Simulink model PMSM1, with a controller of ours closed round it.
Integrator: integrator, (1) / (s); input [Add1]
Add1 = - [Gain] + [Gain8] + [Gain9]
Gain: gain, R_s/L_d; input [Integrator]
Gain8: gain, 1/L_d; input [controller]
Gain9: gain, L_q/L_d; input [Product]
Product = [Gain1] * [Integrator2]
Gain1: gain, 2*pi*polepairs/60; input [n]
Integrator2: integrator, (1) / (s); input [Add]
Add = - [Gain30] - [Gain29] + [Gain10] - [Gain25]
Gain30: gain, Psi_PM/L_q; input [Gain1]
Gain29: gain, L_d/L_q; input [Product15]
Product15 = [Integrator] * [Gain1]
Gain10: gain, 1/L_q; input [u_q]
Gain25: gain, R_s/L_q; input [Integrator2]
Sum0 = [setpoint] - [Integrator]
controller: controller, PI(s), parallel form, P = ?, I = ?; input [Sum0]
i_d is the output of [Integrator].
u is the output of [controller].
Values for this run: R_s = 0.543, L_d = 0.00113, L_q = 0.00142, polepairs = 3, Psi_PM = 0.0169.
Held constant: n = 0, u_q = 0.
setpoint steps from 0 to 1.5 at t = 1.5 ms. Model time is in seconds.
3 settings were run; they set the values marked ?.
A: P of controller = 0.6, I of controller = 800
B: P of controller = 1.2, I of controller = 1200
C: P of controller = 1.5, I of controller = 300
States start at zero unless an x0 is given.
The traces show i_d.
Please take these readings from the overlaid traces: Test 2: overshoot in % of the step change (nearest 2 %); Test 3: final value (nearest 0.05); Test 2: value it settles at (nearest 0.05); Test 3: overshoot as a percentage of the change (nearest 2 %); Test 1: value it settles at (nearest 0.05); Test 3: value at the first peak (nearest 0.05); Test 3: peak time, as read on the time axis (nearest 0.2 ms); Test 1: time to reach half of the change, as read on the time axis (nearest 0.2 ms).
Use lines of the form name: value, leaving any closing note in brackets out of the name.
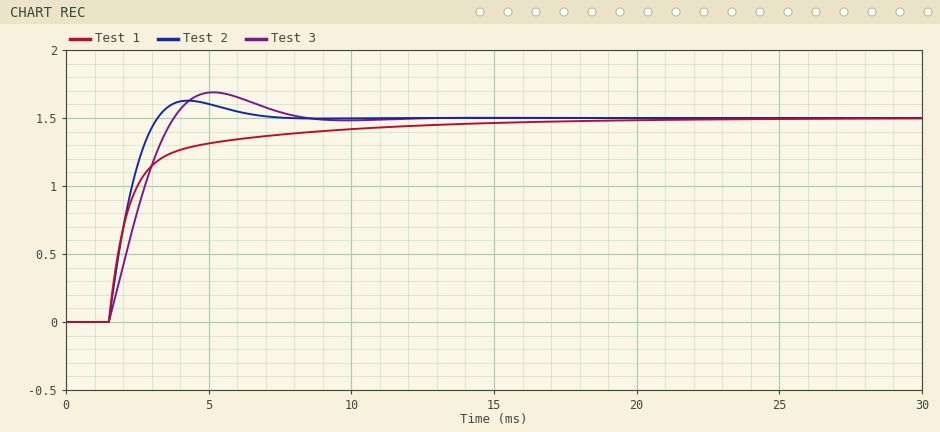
Test 2: overshoot in % of the step change: 8 %
Test 3: final value: 1.50
Test 2: value it settles at: 1.50
Test 3: overshoot as a percentage of the change: 12 %
Test 1: value it settles at: 1.50
Test 3: value at the first peak: 1.70
Test 3: peak time, as read on the time axis: 5.2 ms
Test 1: time to reach half of the change, as read on the time axis: 2.0 ms
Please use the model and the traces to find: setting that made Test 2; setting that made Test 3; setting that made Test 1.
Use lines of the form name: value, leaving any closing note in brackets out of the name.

setting that made Test 2: B
setting that made Test 3: A
setting that made Test 1: C
